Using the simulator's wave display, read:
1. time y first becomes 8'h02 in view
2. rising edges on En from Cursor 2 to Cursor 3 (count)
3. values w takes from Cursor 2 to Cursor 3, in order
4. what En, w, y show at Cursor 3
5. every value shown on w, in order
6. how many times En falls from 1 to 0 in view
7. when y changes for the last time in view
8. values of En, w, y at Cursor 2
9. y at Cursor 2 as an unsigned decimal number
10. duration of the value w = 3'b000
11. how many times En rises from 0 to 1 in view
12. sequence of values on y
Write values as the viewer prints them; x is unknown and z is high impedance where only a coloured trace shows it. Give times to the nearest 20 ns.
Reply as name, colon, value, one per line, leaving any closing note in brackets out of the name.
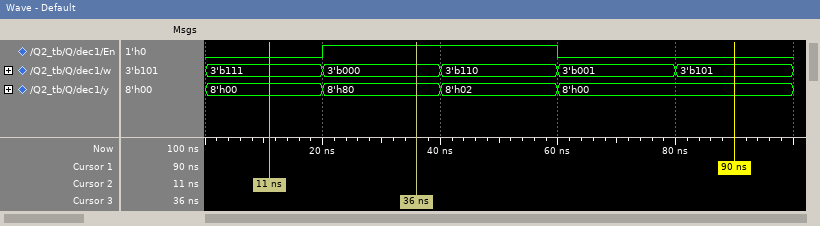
time y first becomes 8'h02 in view: 40 ns
rising edges on En from Cursor 2 to Cursor 3: 1
values w takes from Cursor 2 to Cursor 3, in order: 3'b111, 3'b000
what En, w, y show at Cursor 3: En=1, w=3'b000, y=8'h80
every value shown on w, in order: 3'b111, 3'b000, 3'b110, 3'b001, 3'b101
how many times En falls from 1 to 0 in view: 1
when y changes for the last time in view: 60 ns
values of En, w, y at Cursor 2: En=0, w=3'b111, y=8'h00
y at Cursor 2 as an unsigned decimal number: 0
duration of the value w = 3'b000: 20 ns
how many times En rises from 0 to 1 in view: 1
sequence of values on y: 8'h00, 8'h80, 8'h02, 8'h00
